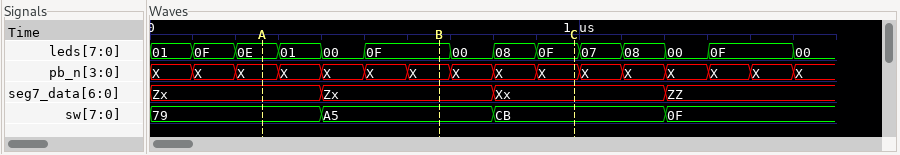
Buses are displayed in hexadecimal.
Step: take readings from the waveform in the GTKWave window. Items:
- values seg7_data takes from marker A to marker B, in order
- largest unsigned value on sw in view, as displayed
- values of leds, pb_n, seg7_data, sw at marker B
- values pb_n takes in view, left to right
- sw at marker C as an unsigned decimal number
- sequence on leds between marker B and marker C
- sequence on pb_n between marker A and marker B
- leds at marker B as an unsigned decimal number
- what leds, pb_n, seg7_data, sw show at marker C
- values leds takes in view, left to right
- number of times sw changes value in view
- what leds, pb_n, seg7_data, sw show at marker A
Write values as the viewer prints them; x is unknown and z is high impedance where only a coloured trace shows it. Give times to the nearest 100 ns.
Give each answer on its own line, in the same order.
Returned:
Zx, Zx
CB
leds=0F, pb_n=X, seg7_data=Zx, sw=A5
X, X, X, X, X, X, X, X, X, X, X, X, X, X, X, X
203
0F, 00, 08, 0F
X, X, X, X, X
15
leds=0F, pb_n=X, seg7_data=Xx, sw=CB
01, 0F, 0E, 01, 00, 0F, 00, 08, 0F, 07, 08, 00, 0F, 00
3
leds=0E, pb_n=X, seg7_data=Zx, sw=79
